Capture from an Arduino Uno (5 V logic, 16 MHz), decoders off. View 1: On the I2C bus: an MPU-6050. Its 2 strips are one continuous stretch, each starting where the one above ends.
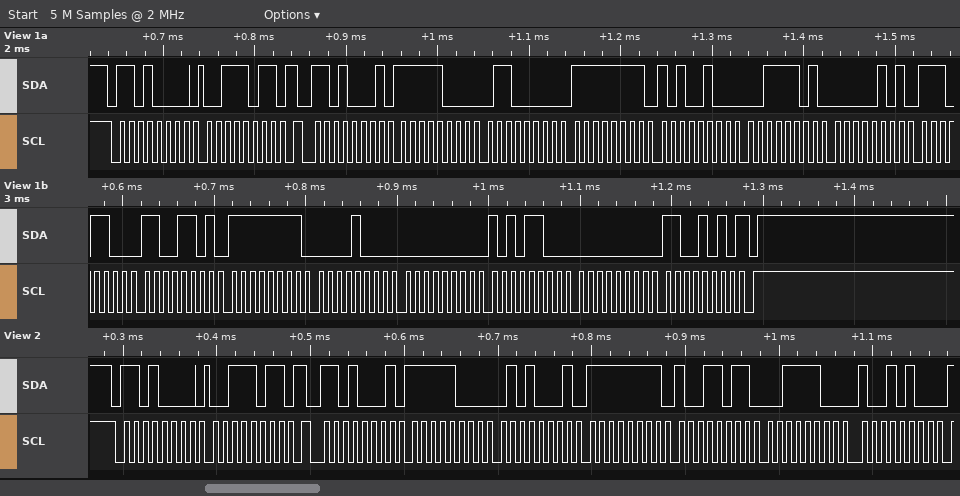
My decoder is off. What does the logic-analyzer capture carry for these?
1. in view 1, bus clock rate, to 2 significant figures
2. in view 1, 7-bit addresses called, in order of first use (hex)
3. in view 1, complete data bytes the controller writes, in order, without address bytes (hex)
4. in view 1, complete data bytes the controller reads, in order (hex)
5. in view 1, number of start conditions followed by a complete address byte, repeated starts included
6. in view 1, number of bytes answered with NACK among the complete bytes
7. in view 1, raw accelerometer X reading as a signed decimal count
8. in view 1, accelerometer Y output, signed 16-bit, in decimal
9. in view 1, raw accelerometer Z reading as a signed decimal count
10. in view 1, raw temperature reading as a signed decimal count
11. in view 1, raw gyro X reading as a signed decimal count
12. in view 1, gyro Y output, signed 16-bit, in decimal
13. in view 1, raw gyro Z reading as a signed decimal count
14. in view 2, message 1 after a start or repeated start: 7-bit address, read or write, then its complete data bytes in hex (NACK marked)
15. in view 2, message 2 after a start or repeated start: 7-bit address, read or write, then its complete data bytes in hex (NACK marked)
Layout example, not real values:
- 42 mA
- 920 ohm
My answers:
- 100 kHz
- 0x68
- 3B
- F8 60 FF A4 3D 05 EC CD FF 08 00 AC 00 CA
- 2
- 1
- -1952
- -92
- 15621
- -4915
- -248
- 172
- 202
- 0x68 write: 3B
- 0x68 read: F8 51 FF 9B 3C 94
